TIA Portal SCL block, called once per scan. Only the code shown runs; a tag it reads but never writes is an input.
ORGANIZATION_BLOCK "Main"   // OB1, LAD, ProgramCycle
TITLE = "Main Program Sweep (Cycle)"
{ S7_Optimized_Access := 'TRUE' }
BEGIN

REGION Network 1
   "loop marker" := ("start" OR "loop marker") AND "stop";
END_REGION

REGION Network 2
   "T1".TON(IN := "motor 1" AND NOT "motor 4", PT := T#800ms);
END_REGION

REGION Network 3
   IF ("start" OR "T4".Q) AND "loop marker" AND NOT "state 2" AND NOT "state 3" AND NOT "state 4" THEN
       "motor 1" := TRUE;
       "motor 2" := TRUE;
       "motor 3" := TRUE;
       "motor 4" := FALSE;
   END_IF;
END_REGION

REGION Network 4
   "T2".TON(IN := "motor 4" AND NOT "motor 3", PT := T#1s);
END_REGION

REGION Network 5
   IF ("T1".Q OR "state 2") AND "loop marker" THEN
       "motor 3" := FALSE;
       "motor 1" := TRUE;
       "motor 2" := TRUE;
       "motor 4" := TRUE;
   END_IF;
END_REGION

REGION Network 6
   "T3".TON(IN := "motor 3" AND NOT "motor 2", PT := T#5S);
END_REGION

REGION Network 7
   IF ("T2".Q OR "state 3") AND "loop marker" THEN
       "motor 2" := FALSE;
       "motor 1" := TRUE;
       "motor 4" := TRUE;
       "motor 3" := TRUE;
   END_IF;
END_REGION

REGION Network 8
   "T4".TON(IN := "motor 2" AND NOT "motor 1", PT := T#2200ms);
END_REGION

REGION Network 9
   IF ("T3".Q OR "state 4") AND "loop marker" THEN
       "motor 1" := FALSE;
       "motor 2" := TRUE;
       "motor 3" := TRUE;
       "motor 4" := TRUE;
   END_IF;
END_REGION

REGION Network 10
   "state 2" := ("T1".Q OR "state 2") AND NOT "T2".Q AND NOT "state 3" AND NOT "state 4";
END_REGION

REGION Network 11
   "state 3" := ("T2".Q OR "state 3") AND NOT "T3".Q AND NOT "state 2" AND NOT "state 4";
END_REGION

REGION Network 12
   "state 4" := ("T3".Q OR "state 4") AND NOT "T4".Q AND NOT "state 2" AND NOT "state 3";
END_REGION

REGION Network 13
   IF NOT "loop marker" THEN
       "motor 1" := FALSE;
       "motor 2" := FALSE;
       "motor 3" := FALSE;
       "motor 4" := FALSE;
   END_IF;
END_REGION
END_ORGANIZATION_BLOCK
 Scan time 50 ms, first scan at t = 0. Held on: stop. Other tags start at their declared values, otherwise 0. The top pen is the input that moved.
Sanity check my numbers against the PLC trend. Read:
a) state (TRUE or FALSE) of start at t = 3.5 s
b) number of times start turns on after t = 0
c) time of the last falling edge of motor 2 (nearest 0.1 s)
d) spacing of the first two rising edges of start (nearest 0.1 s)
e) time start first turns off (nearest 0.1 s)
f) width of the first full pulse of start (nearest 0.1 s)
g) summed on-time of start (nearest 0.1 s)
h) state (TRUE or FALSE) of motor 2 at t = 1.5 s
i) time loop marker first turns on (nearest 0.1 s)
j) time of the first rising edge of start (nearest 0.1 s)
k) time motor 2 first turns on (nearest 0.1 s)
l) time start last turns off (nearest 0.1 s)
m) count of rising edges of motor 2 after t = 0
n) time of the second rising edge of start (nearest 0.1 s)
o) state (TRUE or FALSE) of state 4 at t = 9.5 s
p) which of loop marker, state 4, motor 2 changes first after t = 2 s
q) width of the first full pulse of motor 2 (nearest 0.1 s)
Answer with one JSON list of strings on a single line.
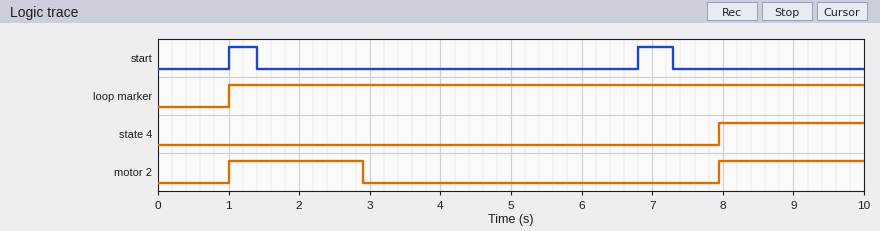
["FALSE", "2", "2.9 s", "5.8 s", "1.4 s", "0.4 s", "0.9 s", "TRUE", "1.0 s", "1.0 s", "1.0 s", "7.3 s", "2", "6.8 s", "TRUE", "motor 2", "1.9 s"]
